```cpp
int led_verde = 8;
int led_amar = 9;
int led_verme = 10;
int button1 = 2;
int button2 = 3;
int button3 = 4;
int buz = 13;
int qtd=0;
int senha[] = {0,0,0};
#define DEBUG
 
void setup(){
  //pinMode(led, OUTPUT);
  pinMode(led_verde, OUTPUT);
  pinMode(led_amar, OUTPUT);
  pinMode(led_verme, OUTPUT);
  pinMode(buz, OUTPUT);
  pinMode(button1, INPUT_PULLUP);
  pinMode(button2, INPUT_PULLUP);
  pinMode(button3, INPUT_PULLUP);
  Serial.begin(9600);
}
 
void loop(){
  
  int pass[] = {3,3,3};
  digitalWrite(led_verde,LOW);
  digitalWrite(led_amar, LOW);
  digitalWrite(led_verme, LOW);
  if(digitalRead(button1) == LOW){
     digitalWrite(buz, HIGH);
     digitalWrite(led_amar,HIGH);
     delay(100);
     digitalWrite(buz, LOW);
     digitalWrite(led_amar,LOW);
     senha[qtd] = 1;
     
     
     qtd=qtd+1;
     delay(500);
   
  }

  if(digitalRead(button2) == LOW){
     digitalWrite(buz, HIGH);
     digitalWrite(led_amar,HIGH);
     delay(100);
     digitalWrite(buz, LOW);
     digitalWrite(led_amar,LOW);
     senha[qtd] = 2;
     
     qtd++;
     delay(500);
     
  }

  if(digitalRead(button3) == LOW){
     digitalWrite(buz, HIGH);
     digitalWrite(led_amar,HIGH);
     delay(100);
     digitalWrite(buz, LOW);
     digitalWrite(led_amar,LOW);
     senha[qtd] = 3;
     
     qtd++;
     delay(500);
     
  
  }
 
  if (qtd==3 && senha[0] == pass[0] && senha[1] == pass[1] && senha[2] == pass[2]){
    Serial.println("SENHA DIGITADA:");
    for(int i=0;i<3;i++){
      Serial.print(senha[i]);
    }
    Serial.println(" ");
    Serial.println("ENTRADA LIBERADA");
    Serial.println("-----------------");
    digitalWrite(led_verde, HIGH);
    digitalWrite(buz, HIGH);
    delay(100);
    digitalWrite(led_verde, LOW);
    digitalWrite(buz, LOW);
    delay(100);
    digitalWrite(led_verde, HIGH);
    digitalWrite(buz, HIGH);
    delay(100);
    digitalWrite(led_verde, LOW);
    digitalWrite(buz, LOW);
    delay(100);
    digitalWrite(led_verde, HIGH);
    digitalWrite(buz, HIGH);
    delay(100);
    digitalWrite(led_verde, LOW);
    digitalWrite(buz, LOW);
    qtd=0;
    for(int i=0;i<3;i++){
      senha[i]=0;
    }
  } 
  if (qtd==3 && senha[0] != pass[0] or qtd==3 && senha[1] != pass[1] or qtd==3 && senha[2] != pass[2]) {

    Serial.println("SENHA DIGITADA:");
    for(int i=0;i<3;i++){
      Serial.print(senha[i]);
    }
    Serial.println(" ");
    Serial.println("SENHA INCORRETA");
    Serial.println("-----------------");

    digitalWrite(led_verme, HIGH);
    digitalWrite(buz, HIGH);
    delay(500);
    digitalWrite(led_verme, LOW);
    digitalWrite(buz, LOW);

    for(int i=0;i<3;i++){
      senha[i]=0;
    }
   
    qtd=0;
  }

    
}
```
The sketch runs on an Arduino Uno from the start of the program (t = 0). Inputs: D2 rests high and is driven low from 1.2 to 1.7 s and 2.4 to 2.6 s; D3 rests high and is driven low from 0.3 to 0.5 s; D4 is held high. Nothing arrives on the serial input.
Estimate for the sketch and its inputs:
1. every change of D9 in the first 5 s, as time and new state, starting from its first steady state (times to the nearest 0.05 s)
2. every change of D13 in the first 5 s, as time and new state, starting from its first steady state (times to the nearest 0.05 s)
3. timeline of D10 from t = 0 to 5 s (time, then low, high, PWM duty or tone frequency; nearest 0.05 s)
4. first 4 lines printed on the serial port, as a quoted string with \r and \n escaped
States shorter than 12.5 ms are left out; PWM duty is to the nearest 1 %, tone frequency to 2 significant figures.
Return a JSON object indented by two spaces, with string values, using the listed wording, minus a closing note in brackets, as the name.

{
  "every change of D9 in the first 5 s, as time and new state, starting from its first steady state": "0 s low; 0.3 s high; 0.4 s low; 1.2 s high; 1.3 s low; 2.4 s high; 2.5 s low",
  "every change of D13 in the first 5 s, as time and new state, starting from its first steady state": "0 s low; 0.3 s high; 0.4 s low; 1.2 s high; 1.3 s low; 2.4 s high; 2.5 s low; 3 s high; 3.5 s low",
  "timeline of D10 from t = 0 to 5 s": "0 s low; 3 s high; 3.5 s low",
  "first 4 lines printed on the serial port, as a quoted string with \\r and \\n escaped": "\"SENHA DIGITADA:\\r\\n211 \\r\\nSENHA INCORRETA\\r\\n-----------------\\r\\n\""
}
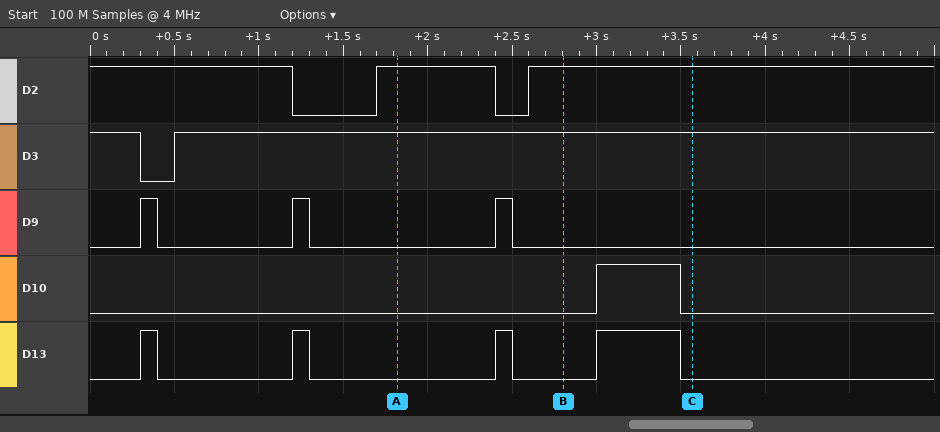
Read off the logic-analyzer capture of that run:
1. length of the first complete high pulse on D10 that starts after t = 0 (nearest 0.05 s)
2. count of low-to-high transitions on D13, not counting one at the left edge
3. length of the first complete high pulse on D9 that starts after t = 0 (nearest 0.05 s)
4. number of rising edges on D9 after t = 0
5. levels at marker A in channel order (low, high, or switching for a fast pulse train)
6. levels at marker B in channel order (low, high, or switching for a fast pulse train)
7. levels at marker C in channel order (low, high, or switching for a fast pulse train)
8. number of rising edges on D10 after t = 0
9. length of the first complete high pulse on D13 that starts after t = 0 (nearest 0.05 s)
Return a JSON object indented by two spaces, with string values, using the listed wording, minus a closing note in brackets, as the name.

{
  "length of the first complete high pulse on D10 that starts after t = 0": "0.50 s",
  "count of low-to-high transitions on D13, not counting one at the left edge": "4",
  "length of the first complete high pulse on D9 that starts after t = 0": "0.10 s",
  "number of rising edges on D9 after t = 0": "3",
  "levels at marker A in channel order": "D2 high, D3 high, D9 low, D10 low, D13 low",
  "levels at marker B in channel order": "D2 high, D3 high, D9 low, D10 low, D13 low",
  "levels at marker C in channel order": "D2 high, D3 high, D9 low, D10 low, D13 low",
  "number of rising edges on D10 after t = 0": "1",
  "length of the first complete high pulse on D13 that starts after t = 0": "0.10 s"
}
